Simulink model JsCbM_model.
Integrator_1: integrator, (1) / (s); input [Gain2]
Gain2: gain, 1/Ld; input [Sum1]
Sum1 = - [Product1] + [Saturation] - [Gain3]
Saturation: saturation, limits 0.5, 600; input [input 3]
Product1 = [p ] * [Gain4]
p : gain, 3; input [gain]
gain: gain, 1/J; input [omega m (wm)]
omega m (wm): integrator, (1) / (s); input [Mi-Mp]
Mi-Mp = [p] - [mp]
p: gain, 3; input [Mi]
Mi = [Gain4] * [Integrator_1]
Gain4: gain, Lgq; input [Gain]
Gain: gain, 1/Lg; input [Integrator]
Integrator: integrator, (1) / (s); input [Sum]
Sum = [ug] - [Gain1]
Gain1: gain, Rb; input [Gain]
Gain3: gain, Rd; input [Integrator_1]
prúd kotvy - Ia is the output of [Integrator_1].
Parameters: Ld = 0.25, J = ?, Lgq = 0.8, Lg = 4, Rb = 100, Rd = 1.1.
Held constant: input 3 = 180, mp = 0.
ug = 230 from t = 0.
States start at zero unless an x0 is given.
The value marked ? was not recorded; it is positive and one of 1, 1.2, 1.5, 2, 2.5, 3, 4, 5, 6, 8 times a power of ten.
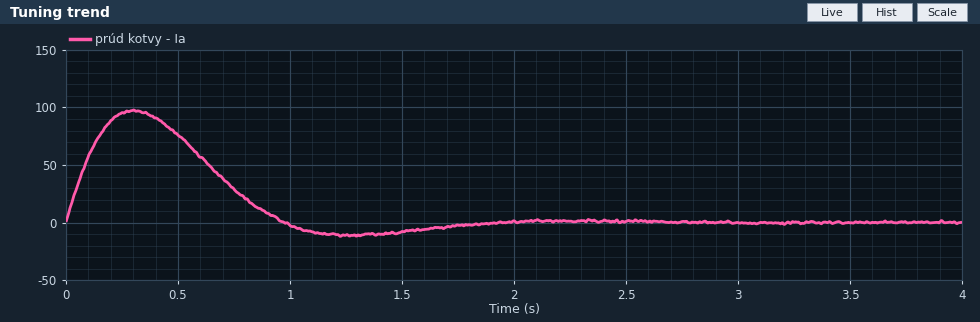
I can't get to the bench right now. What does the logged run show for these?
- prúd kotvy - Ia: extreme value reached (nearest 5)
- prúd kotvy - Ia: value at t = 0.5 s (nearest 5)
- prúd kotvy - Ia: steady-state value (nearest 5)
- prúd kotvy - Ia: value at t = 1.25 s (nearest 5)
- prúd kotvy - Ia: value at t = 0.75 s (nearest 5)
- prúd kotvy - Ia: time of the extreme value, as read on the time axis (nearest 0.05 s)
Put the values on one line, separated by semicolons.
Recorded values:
95; 75; 0; -10; 30; 0.30 s
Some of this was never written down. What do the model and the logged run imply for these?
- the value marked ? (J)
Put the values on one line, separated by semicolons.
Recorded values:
8
